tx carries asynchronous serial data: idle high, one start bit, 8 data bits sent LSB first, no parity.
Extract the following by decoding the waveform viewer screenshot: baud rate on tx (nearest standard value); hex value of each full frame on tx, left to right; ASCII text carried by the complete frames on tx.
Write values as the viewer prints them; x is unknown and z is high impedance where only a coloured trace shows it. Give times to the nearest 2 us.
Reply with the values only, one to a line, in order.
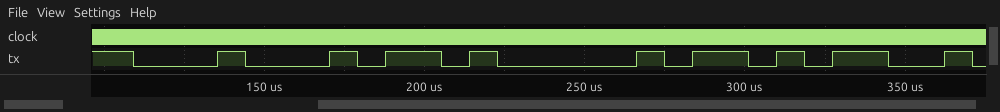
115200 baud
44, 41
"DA"
